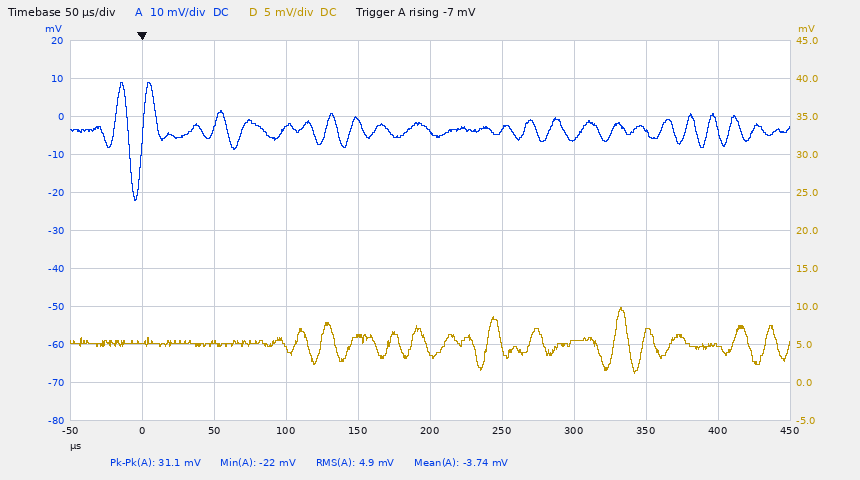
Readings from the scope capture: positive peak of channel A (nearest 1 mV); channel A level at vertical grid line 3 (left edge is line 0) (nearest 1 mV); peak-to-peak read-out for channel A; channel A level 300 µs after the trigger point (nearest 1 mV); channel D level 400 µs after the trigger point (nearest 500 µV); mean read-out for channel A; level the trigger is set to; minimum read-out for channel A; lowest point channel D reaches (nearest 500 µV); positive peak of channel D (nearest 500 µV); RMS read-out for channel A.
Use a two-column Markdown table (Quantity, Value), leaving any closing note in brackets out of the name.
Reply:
| Quantity | Value |
|---|---|
| positive peak of channel A | 9 mV |
| channel A level at vertical grid line 3 (left edge is line 0) | -3 mV |
| peak-to-peak read-out for channel A | 31.1 mV |
| channel A level 300 µs after the trigger point | -6 mV |
| channel D level 400 µs after the trigger point | 5.0 mV |
| mean read-out for channel A | -3.74 mV |
| level the trigger is set to | -7 mV |
| minimum read-out for channel A | -22 mV |
| lowest point channel D reaches | 1.0 mV |
| positive peak of channel D | 10.0 mV |
| RMS read-out for channel A | 4.9 mV |
